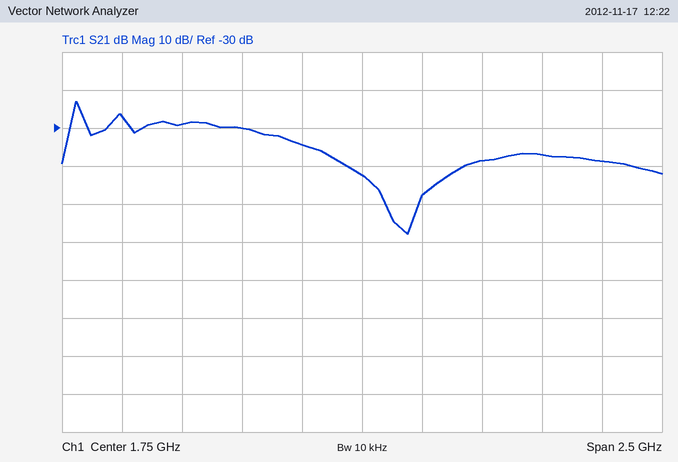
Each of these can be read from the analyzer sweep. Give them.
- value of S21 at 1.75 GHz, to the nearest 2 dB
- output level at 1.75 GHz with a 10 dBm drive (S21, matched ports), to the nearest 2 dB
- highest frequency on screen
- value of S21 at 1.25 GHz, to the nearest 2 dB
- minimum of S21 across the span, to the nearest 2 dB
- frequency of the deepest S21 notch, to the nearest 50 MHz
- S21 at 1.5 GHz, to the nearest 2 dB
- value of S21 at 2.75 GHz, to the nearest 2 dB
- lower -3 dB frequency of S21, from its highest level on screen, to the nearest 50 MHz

-42 dB
-32 dBm
3 GHz
-30 dB
-58 dB
1.95 GHz
-34 dB
-38 dB
550 MHz
